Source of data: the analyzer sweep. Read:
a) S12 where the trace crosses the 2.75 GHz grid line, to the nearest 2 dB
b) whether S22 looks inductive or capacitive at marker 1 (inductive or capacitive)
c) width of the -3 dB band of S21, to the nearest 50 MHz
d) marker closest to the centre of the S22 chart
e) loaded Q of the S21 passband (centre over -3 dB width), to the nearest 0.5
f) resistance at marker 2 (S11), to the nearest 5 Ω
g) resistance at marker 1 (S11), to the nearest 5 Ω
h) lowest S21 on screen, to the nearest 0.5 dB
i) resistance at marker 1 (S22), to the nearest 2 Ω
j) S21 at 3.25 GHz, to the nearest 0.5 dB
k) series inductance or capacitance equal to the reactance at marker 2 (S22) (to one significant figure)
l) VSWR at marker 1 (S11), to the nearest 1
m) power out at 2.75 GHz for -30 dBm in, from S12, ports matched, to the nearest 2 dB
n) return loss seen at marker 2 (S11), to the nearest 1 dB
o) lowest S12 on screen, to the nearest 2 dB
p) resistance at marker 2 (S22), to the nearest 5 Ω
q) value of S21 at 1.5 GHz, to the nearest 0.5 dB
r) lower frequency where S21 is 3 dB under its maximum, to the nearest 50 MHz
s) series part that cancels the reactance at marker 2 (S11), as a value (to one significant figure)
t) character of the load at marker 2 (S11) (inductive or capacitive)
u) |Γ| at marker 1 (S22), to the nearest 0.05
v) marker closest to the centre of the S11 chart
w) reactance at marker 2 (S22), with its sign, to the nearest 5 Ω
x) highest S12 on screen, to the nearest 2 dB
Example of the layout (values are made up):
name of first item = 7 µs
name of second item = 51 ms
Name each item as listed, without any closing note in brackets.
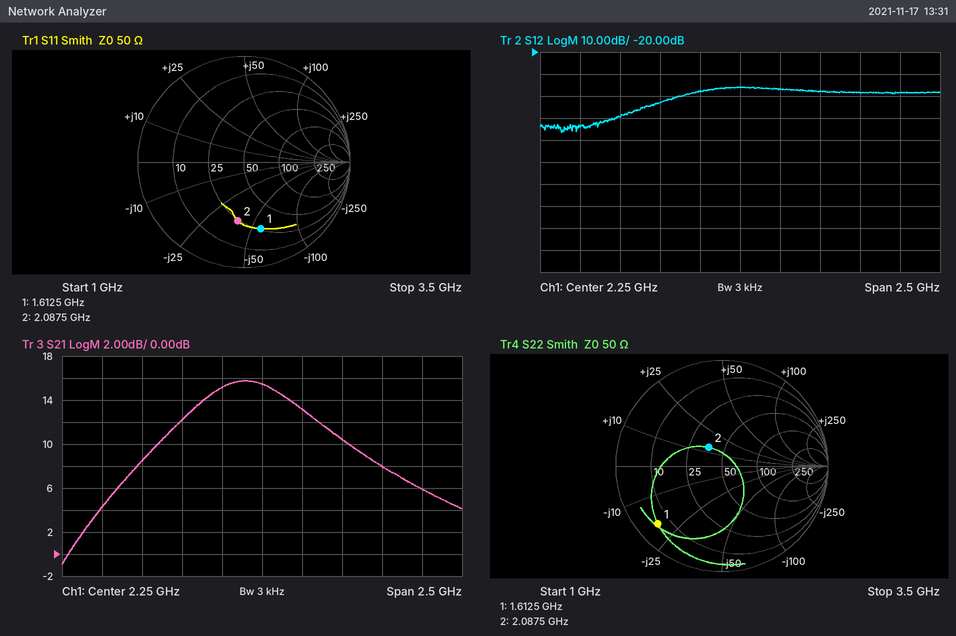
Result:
S12 where the trace crosses the 2.75 GHz grid line, to the nearest 2 dB = -38 dB
whether S22 looks inductive or capacitive at marker 1 = capacitive
width of the -3 dB band of S21, to the nearest 50 MHz = 750 MHz
marker closest to the centre of the S22 chart = marker 2
loaded Q of the S21 passband (centre over -3 dB width), to the nearest 0.5 = 3.0
resistance at marker 2 (S11), to the nearest 5 Ω = 25 Ω
resistance at marker 1 (S11), to the nearest 5 Ω = 25 Ω
lowest S21 on screen, to the nearest 0.5 dB = -1.0 dB
resistance at marker 1 (S22), to the nearest 2 Ω = 6 Ω
S21 at 3.25 GHz, to the nearest 0.5 dB = 6.0 dB
series inductance or capacitance equal to the reactance at marker 2 (S22) = 1 nH
VSWR at marker 1 (S11), to the nearest 1 = 5
power out at 2.75 GHz for -30 dBm in, from S12, ports matched, to the nearest 2 dB = -68 dBm
return loss seen at marker 2 (S11), to the nearest 1 dB = 5 dB
lowest S12 on screen, to the nearest 2 dB = -56 dB
resistance at marker 2 (S22), to the nearest 5 Ω = 35 Ω
value of S21 at 1.5 GHz, to the nearest 0.5 dB = 8.5 dB
lower frequency where S21 is 3 dB under its maximum, to the nearest 50 MHz = 1.80 GHz
series part that cancels the reactance at marker 2 (S11), as a value = 3 nH
character of the load at marker 2 (S11) = capacitive
|Γ| at marker 1 (S22), to the nearest 0.05 = 0.80
marker closest to the centre of the S11 chart = marker 2
reactance at marker 2 (S22), with its sign, to the nearest 5 Ω = +15 Ω
highest S12 on screen, to the nearest 2 dB = -36 dB
